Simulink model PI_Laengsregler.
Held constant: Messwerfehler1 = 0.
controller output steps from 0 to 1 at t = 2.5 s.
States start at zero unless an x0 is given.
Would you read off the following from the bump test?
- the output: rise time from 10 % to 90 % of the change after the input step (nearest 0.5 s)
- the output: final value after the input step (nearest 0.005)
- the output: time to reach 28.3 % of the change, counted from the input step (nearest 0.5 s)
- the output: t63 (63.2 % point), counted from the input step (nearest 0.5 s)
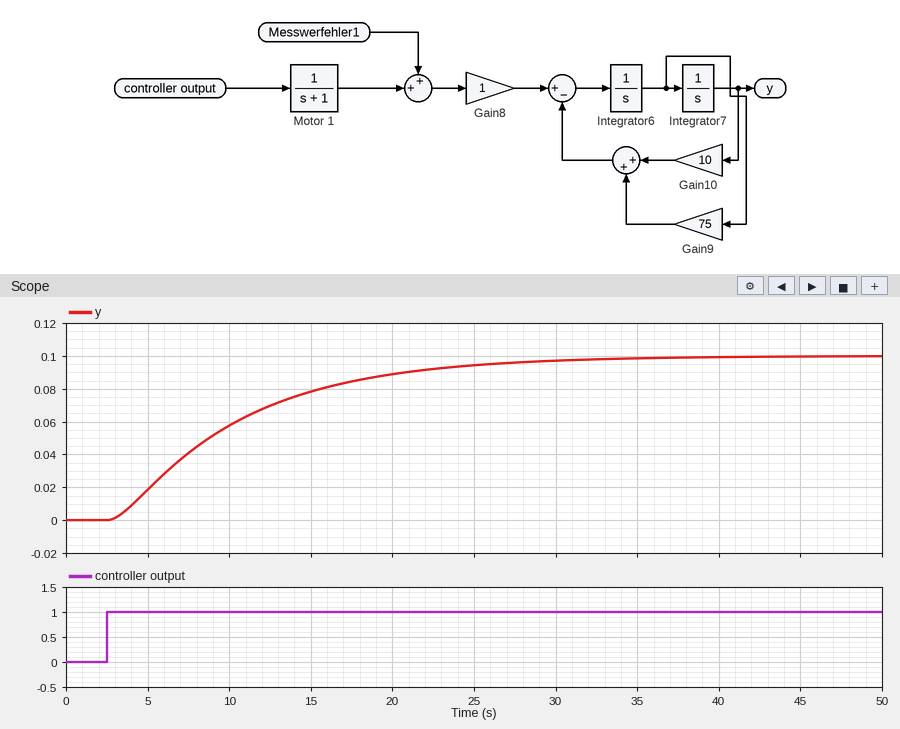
16.5 s
0.100
3.5 s
8.5 s
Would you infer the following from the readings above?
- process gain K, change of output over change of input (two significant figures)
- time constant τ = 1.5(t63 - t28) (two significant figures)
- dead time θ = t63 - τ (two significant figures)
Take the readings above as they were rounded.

0.10
7.5 s
1.0 s
